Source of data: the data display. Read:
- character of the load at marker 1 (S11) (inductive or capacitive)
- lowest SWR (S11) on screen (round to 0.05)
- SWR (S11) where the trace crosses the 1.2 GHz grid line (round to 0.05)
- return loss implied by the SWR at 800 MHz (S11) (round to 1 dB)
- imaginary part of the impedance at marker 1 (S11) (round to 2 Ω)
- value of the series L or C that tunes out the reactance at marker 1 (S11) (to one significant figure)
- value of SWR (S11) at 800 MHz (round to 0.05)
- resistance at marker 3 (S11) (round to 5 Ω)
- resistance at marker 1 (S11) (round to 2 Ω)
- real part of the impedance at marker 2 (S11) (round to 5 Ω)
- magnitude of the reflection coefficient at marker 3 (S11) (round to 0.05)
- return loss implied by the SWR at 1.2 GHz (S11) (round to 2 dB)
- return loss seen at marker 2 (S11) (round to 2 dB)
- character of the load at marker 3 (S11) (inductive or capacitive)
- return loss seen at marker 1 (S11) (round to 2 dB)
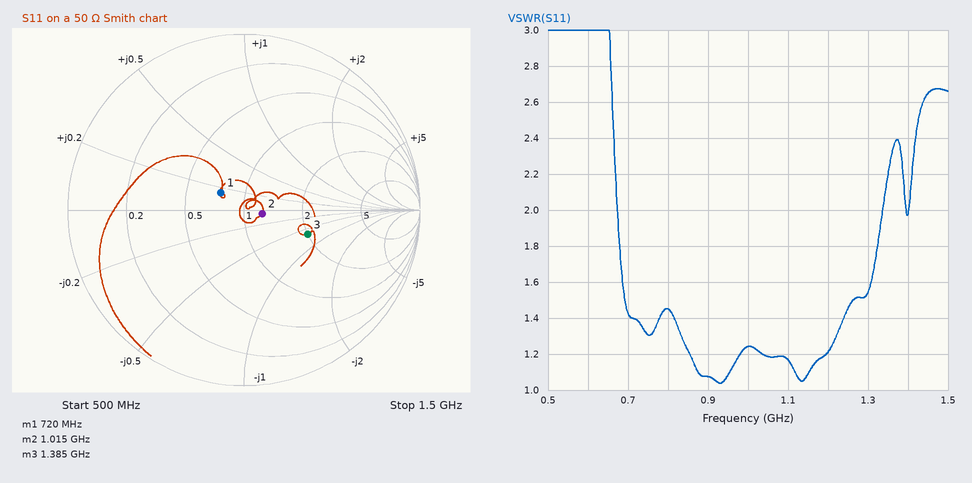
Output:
inductive
1.05
1.20
15 dB
+8 Ω
30 pF
1.45
100 Ω
38 Ω
60 Ω
0.40
20 dB
20 dB
capacitive
16 dB
